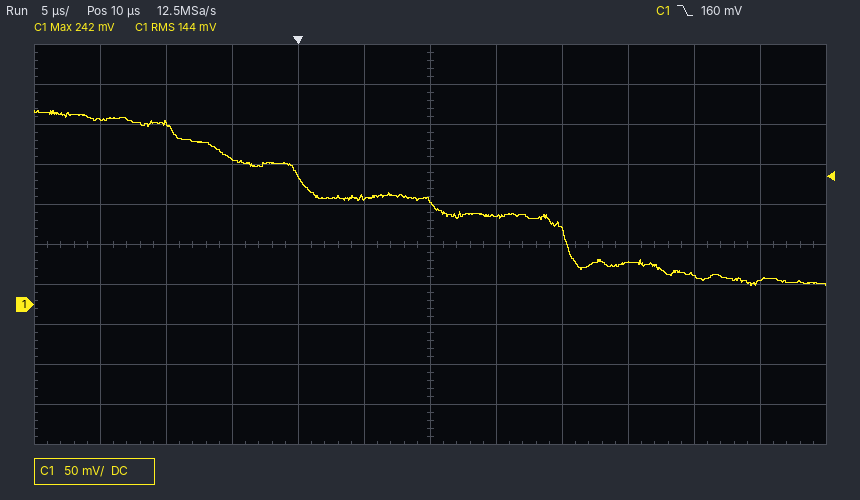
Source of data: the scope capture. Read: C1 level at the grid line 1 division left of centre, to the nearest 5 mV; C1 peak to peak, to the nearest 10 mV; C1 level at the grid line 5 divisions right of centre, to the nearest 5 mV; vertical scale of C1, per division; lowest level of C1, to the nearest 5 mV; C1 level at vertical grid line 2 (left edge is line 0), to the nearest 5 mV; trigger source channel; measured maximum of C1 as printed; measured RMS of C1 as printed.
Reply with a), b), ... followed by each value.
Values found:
a) 135 mV
b) 220 mV
c) 30 mV
d) 50 mV
e) 25 mV
f) 225 mV
g) C1
h) 242 mV
i) 144 mV
